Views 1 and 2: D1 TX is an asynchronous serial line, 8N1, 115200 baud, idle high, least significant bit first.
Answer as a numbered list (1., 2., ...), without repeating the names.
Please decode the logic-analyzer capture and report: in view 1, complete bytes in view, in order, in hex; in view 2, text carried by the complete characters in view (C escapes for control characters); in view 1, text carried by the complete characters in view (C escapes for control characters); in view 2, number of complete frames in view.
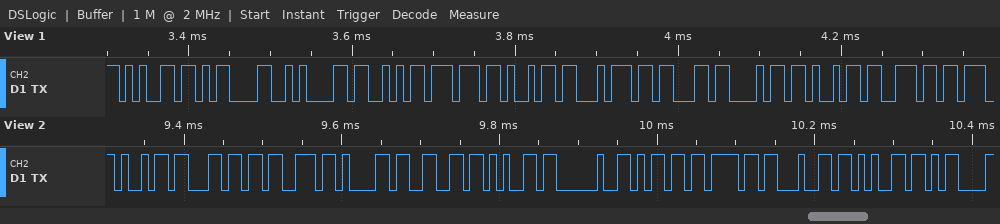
1. 65 0D 0A 53 77 69 74 63 68 69 6E
2. "ilsafe mode\r"
3. "e\r\nSwitchin"
4. 12
